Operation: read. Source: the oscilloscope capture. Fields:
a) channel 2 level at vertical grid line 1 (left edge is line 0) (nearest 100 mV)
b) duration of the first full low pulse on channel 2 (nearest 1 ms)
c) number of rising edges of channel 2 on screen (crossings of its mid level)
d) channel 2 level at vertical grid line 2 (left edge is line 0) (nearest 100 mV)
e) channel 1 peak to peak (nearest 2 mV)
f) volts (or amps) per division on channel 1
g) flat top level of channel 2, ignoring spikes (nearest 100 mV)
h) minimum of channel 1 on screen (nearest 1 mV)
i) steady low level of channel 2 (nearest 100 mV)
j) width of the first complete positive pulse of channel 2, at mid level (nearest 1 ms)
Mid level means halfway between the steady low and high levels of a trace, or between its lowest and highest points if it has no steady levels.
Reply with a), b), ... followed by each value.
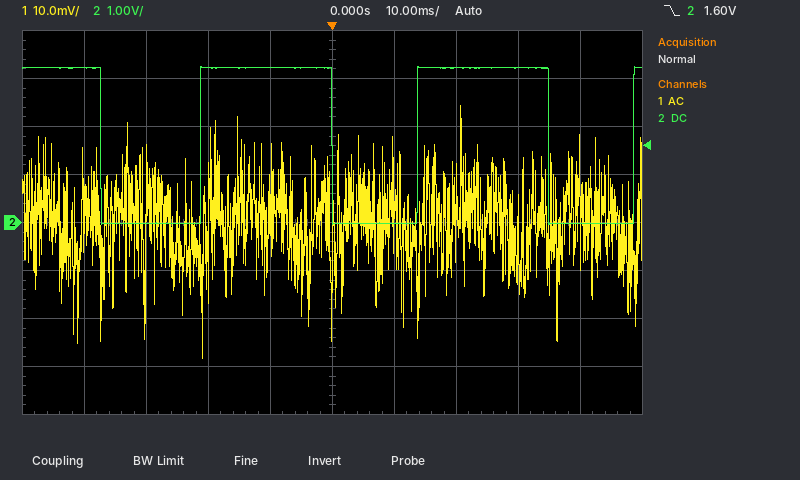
a) 3.2 V
b) 16 ms
c) 3
d) 0.0 V
e) 52 mV
f) 10 mV
g) 3.2 V
h) -28 mV
i) 0.0 V
j) 21 ms
